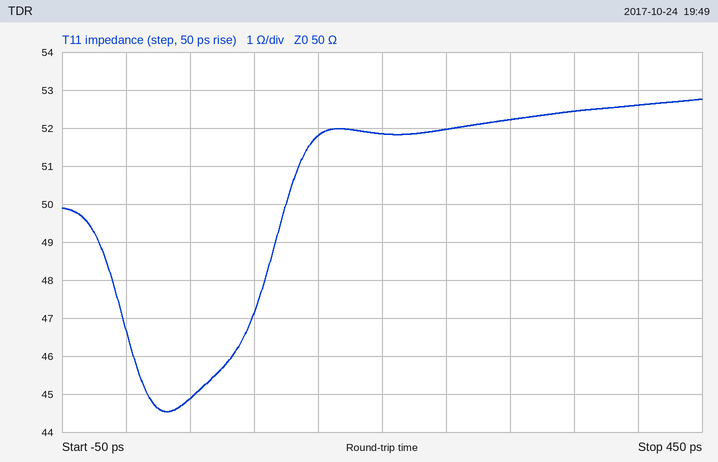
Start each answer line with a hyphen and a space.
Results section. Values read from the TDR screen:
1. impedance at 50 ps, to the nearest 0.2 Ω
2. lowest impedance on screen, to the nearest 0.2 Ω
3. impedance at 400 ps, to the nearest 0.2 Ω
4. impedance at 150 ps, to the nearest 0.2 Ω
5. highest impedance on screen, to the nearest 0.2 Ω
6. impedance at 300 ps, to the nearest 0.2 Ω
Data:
- 44.8 Ω
- 44.6 Ω
- 52.6 Ω
- 51.8 Ω
- 52.8 Ω
- 52.2 Ω
